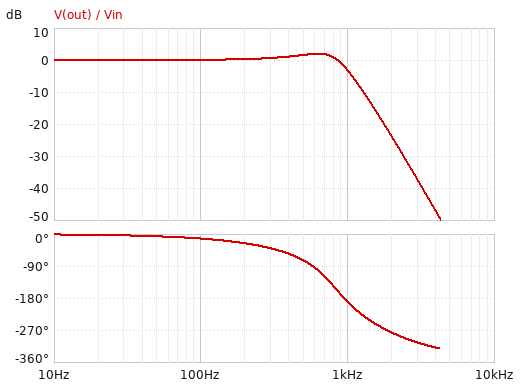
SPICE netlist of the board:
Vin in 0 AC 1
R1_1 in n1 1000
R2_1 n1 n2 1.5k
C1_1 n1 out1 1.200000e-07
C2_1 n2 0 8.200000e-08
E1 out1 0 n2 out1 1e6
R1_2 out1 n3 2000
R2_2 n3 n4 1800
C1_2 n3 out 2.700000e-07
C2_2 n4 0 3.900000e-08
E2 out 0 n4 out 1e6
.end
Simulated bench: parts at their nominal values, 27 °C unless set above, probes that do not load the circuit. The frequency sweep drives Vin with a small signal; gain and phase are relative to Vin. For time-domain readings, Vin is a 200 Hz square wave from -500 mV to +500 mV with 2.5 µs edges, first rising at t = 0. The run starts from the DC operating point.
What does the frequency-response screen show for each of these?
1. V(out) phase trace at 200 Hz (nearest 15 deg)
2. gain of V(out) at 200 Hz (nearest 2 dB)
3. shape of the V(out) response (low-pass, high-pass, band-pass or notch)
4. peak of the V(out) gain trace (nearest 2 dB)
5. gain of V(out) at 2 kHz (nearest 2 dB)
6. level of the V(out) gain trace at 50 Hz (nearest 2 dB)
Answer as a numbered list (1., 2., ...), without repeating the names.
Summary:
1. -30 deg
2. 0 dB
3. low-pass
4. 2 dB
5. -24 dB
6. 0 dB
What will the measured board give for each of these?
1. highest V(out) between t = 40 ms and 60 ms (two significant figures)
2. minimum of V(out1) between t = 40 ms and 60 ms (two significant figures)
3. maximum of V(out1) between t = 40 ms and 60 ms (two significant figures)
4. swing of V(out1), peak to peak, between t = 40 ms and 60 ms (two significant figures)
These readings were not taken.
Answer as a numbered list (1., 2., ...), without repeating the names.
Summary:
1. 720 mV
2. -510 mV
3. 510 mV
4. 1.0 V
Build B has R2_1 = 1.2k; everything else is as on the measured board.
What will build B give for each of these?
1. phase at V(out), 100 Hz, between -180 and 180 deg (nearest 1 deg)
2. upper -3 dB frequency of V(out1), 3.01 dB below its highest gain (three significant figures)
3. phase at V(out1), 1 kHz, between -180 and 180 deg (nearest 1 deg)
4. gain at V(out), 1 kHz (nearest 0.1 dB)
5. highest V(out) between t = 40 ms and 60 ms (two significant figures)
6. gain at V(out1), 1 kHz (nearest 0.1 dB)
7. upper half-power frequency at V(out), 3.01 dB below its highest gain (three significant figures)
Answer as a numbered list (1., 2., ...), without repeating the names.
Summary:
1. -12 deg
2. 1.22 kHz
3. -65 deg
4. -2.4 dB
5. 740 mV
6. -2.0 dB
7. 924 Hz
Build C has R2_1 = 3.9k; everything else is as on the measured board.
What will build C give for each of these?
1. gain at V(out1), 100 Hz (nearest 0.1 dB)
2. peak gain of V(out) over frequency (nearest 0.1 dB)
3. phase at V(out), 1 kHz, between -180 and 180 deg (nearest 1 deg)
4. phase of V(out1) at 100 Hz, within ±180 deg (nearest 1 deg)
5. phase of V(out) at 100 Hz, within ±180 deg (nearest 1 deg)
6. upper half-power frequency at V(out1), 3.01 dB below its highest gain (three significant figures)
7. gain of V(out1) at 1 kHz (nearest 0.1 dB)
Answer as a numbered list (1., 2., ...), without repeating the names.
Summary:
1. -0.1 dB
2. 0 dB
3. 140 deg
4. -14 deg
5. -20 deg
6. 505 Hz
7. -8.2 dB
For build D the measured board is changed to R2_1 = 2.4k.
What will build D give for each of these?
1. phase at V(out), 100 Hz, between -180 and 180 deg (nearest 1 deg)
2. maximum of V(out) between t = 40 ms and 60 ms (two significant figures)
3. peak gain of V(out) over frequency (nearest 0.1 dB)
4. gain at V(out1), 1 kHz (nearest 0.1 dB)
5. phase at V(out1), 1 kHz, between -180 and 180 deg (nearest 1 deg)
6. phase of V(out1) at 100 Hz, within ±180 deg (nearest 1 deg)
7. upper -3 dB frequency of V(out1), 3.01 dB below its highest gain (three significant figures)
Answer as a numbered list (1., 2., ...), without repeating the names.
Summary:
1. -15 deg
2. 670 mV
3. 0.9 dB
4. -4.9 dB
5. -88 deg
6. -10 deg
7. 764 Hz
